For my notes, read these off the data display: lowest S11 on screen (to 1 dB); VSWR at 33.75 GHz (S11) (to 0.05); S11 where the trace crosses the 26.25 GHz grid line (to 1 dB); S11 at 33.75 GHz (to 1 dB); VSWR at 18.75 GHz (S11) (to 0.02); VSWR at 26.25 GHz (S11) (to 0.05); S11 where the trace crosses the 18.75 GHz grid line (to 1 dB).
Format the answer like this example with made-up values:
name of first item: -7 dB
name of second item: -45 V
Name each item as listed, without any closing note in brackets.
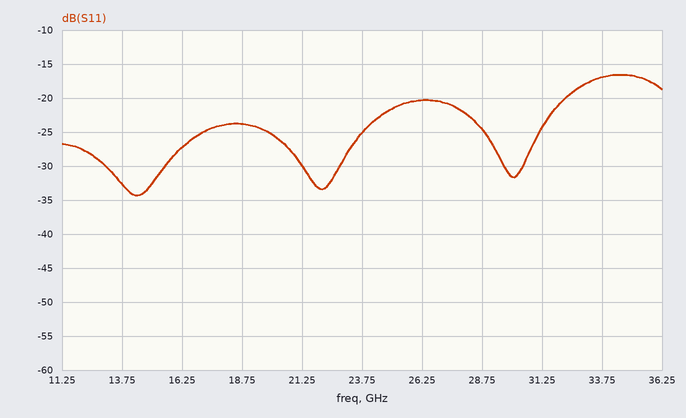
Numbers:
lowest S11 on screen: -34 dB
VSWR at 33.75 GHz (S11): 1.35
S11 where the trace crosses the 26.25 GHz grid line: -20 dB
S11 at 33.75 GHz: -17 dB
VSWR at 18.75 GHz (S11): 1.14
VSWR at 26.25 GHz (S11): 1.20
S11 where the trace crosses the 18.75 GHz grid line: -24 dB
